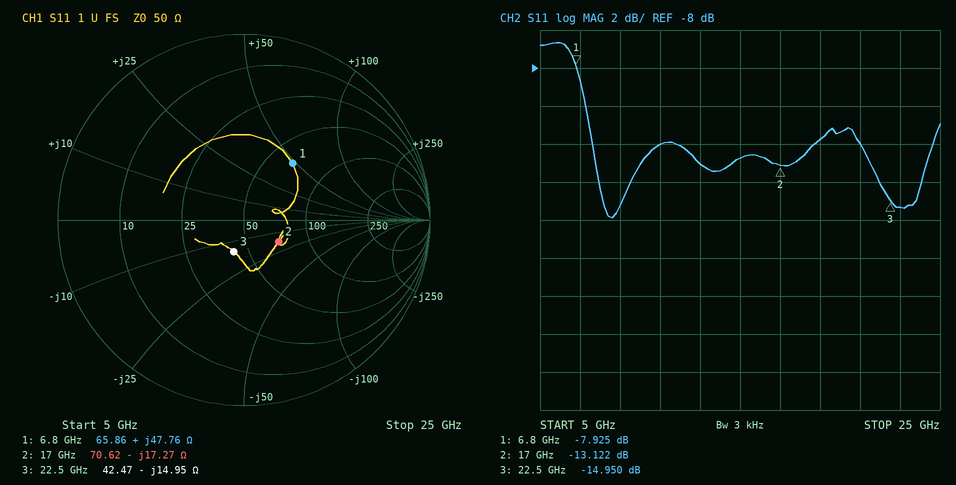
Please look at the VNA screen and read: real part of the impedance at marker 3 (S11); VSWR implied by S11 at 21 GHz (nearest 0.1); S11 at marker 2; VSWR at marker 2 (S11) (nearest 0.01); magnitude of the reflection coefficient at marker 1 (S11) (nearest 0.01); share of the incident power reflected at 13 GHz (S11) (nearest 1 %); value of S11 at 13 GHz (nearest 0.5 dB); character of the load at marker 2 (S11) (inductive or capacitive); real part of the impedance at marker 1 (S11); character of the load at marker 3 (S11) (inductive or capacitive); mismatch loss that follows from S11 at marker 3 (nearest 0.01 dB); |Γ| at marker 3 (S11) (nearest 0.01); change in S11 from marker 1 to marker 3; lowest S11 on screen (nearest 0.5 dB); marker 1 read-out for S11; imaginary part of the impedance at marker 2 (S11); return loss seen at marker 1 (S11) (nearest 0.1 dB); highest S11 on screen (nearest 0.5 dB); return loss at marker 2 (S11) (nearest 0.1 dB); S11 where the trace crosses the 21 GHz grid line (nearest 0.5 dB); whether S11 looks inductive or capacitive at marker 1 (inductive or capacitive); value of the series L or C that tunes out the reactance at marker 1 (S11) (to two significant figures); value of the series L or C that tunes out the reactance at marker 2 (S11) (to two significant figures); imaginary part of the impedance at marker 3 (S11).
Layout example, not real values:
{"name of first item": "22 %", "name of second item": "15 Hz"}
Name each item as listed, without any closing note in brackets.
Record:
{"real part of the impedance at marker 3": "42.47 Ω", "VSWR implied by S11 at 21 GHz": "1.7", "S11 at marker 2": "-13.122 dB", "VSWR at marker 2 (S11)": "1.57", "magnitude of the reflection coefficient at marker 1 (S11)": "0.40", "share of the incident power reflected at 13 GHz (S11)": "5 %", "value of S11 at 13 GHz": "-13.0 dB", "character of the load at marker 2 (S11)": "capacitive", "real part of the impedance at marker 1": "65.86 Ω", "character of the load at marker 3 (S11)": "capacitive", "mismatch loss that follows from S11 at marker 3": "0.14 dB", "|Γ| at marker 3 (S11)": "0.18", "change in S11 from marker 1 to marker 3": "-7.025 dB", "lowest S11 on screen": "-16.0 dB", "marker 1 read-out for S11": "-7.925 dB", "imaginary part of the impedance at marker 2": "-17.27 Ω", "return loss seen at marker 1 (S11)": "7.9 dB", "highest S11 on screen": "-6.5 dB", "return loss at marker 2 (S11)": "13.1 dB", "S11 where the trace crosses the 21 GHz grid line": "-12.0 dB", "whether S11 looks inductive or capacitive at marker 1": "inductive", "value of the series L or C that tunes out the reactance at marker 1 (S11)": "490 fF", "value of the series L or C that tunes out the reactance at marker 2 (S11)": "160 pH", "imaginary part of the impedance at marker 3": "-14.95 Ω"}
